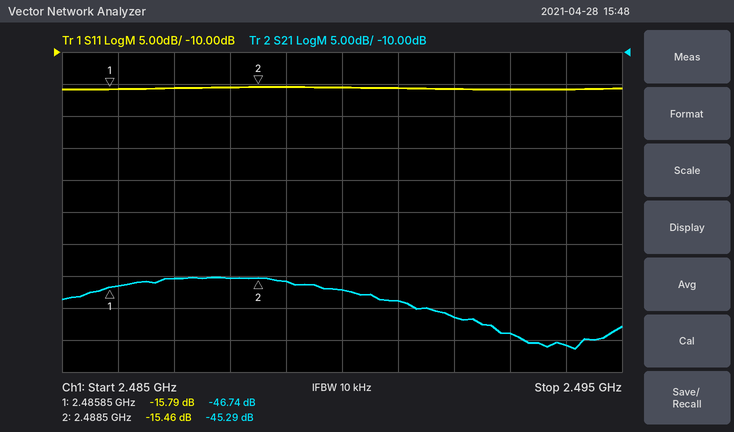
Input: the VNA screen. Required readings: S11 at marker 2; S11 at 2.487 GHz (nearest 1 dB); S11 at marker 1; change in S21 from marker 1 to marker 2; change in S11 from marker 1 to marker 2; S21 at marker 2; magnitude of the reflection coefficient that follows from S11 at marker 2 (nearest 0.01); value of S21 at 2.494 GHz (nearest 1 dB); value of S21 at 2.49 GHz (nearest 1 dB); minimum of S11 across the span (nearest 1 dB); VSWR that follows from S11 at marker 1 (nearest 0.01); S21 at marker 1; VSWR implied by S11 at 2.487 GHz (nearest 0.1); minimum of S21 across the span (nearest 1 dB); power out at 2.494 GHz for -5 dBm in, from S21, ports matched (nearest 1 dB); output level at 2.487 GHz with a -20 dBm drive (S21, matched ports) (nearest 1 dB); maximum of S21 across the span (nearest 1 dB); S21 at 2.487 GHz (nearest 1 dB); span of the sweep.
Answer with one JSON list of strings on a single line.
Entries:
["-15.46 dB", "-16 dB", "-15.79 dB", "1.45 dB", "0.33 dB", "-45.29 dB", "0.17", "-56 dB", "-47 dB", "-16 dB", "1.39", "-46.74 dB", "1.4", "-56 dB", "-61 dBm", "-65 dBm", "-45 dB", "-45 dB", "10 MHz"]
